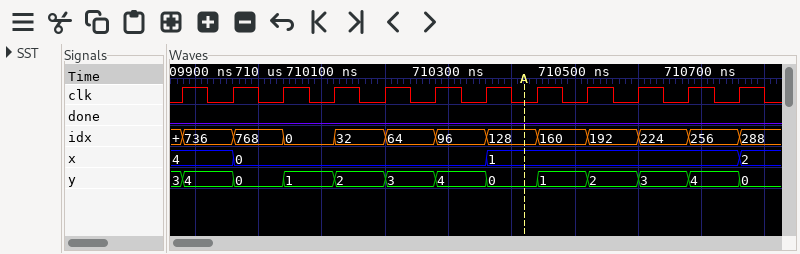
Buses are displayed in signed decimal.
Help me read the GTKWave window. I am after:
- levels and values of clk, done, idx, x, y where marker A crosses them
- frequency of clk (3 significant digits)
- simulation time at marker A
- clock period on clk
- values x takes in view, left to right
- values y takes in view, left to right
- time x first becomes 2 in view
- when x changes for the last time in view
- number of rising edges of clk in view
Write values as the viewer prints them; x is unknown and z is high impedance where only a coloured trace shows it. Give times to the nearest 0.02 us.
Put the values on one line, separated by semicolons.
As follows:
clk=0, done=0, idx=128, x=1, y=0; 12.5 MHz; 710.42 us; 0.08 us; 4, 0, 1, 2; 3, 4, 0, 1, 2, 3, 4, 0, 1, 2, 3, 4, 0; 710.76 us; 710.76 us; 12
